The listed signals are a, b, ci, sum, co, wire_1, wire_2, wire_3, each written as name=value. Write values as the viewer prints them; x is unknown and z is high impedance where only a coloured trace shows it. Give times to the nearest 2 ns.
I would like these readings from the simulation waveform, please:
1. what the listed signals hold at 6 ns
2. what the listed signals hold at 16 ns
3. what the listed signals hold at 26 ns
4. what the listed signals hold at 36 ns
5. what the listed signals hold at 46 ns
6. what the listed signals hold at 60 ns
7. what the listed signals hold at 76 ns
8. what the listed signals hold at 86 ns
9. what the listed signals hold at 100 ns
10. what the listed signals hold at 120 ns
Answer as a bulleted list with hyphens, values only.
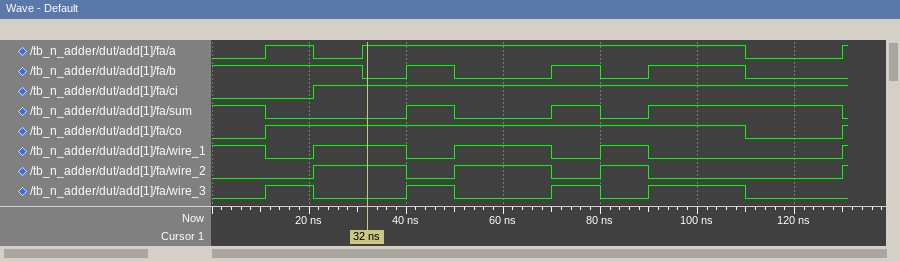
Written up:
- a=0, b=1, ci=0, sum=1, co=0, wire_1=1, wire_2=0, wire_3=0
- a=1, b=1, ci=0, sum=0, co=1, wire_1=0, wire_2=0, wire_3=1
- a=0, b=1, ci=1, sum=0, co=1, wire_1=1, wire_2=1, wire_3=0
- a=1, b=0, ci=1, sum=0, co=1, wire_1=1, wire_2=1, wire_3=0
- a=1, b=1, ci=1, sum=1, co=1, wire_1=0, wire_2=0, wire_3=1
- a=1, b=0, ci=1, sum=0, co=1, wire_1=1, wire_2=1, wire_3=0
- a=1, b=1, ci=1, sum=1, co=1, wire_1=0, wire_2=0, wire_3=1
- a=1, b=0, ci=1, sum=0, co=1, wire_1=1, wire_2=1, wire_3=0
- a=1, b=1, ci=1, sum=1, co=1, wire_1=0, wire_2=0, wire_3=1
- a=0, b=0, ci=1, sum=1, co=0, wire_1=0, wire_2=0, wire_3=0
